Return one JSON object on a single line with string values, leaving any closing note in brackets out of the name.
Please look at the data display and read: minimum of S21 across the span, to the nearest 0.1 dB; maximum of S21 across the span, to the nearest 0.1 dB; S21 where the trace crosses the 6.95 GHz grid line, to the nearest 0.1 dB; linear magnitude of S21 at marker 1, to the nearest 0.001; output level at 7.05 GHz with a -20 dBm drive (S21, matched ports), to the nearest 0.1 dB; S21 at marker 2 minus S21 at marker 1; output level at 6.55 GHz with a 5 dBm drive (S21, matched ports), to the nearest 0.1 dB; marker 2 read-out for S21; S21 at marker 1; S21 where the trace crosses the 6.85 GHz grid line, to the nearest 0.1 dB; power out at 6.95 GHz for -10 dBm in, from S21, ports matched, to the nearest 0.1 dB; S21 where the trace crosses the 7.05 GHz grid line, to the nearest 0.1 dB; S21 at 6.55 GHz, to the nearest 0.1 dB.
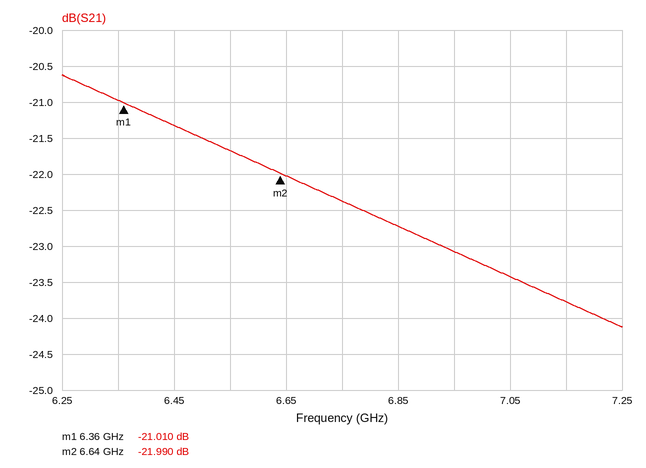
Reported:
{"minimum of S21 across the span, to the nearest 0.1 dB": "-24.1 dB", "maximum of S21 across the span, to the nearest 0.1 dB": "-20.6 dB", "S21 where the trace crosses the 6.95 GHz grid line, to the nearest 0.1 dB": "-23.1 dB", "linear magnitude of S21 at marker 1, to the nearest 0.001": "0.089", "output level at 7.05 GHz with a -20 dBm drive (S21, matched ports), to the nearest 0.1 dB": "-43.4 dBm", "S21 at marker 2 minus S21 at marker 1": "-0.980 dB", "output level at 6.55 GHz with a 5 dBm drive (S21, matched ports), to the nearest 0.1 dB": "-16.7 dBm", "marker 2 read-out for S21": "-21.990 dB", "S21 at marker 1": "-21.010 dB", "S21 where the trace crosses the 6.85 GHz grid line, to the nearest 0.1 dB": "-22.7 dB", "power out at 6.95 GHz for -10 dBm in, from S21, ports matched, to the nearest 0.1 dB": "-33.1 dBm", "S21 where the trace crosses the 7.05 GHz grid line, to the nearest 0.1 dB": "-23.4 dB", "S21 at 6.55 GHz, to the nearest 0.1 dB": "-21.7 dB"}
